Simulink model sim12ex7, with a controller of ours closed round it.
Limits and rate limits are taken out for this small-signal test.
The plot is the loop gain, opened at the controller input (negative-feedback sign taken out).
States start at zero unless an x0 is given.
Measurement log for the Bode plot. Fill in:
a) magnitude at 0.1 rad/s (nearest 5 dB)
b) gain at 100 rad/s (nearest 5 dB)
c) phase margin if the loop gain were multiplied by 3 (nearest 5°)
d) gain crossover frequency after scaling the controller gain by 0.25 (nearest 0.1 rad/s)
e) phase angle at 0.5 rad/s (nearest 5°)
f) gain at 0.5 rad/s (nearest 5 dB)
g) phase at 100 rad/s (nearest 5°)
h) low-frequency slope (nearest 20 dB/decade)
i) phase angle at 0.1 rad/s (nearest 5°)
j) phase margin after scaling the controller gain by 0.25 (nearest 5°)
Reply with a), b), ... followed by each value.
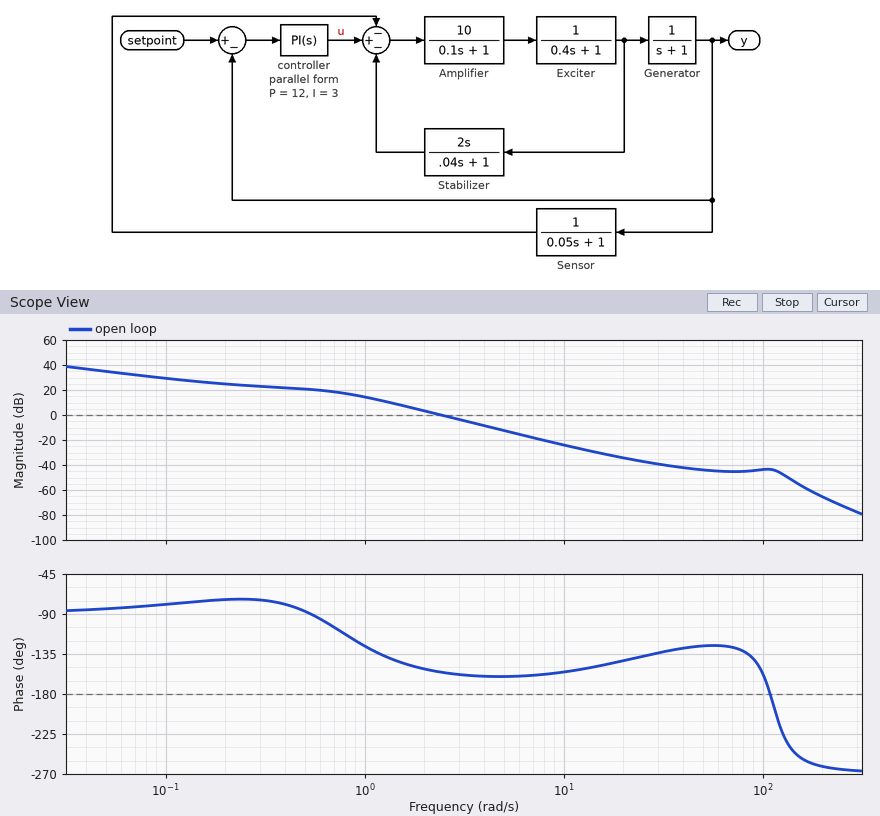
a) 30 dB
b) -45 dB
c) 20°
d) 1.2 rad/s
e) -85°
f) 20 dB
g) -155°
h) -20 dB/decade
i) -80°
j) 45°
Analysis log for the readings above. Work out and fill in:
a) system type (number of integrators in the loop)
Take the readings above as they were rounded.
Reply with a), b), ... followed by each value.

a) 1
